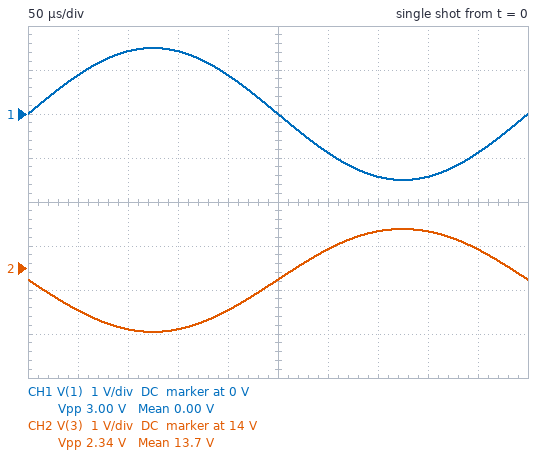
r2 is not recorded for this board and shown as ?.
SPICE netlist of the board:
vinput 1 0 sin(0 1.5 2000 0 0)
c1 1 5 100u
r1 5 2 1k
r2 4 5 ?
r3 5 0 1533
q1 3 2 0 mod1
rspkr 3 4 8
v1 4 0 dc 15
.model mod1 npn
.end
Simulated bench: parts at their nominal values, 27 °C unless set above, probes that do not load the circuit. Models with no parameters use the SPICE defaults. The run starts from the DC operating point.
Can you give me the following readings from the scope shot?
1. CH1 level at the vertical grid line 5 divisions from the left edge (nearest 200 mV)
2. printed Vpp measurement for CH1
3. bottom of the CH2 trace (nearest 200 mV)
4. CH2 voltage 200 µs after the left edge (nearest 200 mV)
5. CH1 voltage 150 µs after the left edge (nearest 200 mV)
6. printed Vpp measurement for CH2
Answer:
0 V
3.00 V
12.6 V
13.0 V
1.4 V
2.34 V
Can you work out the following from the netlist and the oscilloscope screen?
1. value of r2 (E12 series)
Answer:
3.9 kΩ
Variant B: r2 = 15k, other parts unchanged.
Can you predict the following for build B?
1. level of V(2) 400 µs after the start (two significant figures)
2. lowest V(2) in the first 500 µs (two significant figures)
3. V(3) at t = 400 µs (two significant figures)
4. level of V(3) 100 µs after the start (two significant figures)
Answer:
-350 mV
-420 mV
15 V
14 V
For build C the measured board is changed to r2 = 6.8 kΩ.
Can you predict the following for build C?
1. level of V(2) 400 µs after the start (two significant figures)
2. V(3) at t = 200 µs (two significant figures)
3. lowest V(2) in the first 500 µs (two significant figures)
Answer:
290 mV
14 V
220 mV
